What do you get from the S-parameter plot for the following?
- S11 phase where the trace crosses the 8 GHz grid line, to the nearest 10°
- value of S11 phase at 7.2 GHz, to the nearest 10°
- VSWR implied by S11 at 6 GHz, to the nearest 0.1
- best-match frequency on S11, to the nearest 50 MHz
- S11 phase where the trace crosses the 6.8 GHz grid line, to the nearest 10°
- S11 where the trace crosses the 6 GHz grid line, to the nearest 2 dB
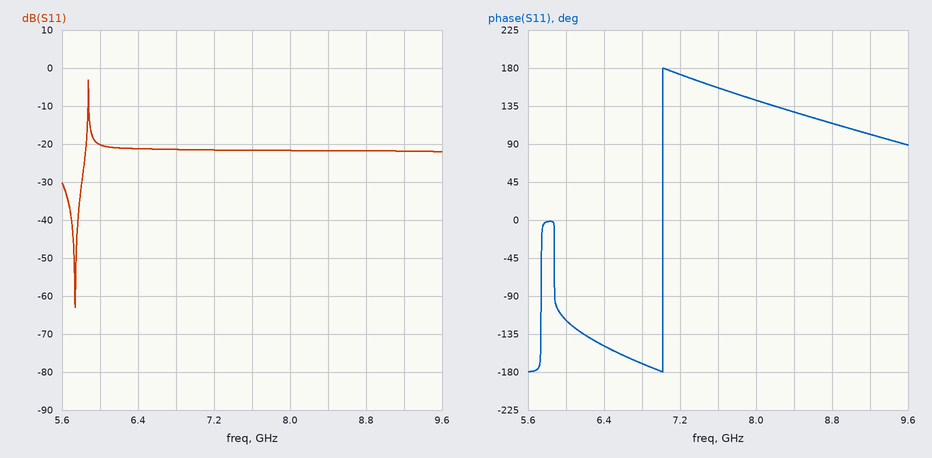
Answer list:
140°
170°
1.2
5.75 GHz
-170°
-20 dB
